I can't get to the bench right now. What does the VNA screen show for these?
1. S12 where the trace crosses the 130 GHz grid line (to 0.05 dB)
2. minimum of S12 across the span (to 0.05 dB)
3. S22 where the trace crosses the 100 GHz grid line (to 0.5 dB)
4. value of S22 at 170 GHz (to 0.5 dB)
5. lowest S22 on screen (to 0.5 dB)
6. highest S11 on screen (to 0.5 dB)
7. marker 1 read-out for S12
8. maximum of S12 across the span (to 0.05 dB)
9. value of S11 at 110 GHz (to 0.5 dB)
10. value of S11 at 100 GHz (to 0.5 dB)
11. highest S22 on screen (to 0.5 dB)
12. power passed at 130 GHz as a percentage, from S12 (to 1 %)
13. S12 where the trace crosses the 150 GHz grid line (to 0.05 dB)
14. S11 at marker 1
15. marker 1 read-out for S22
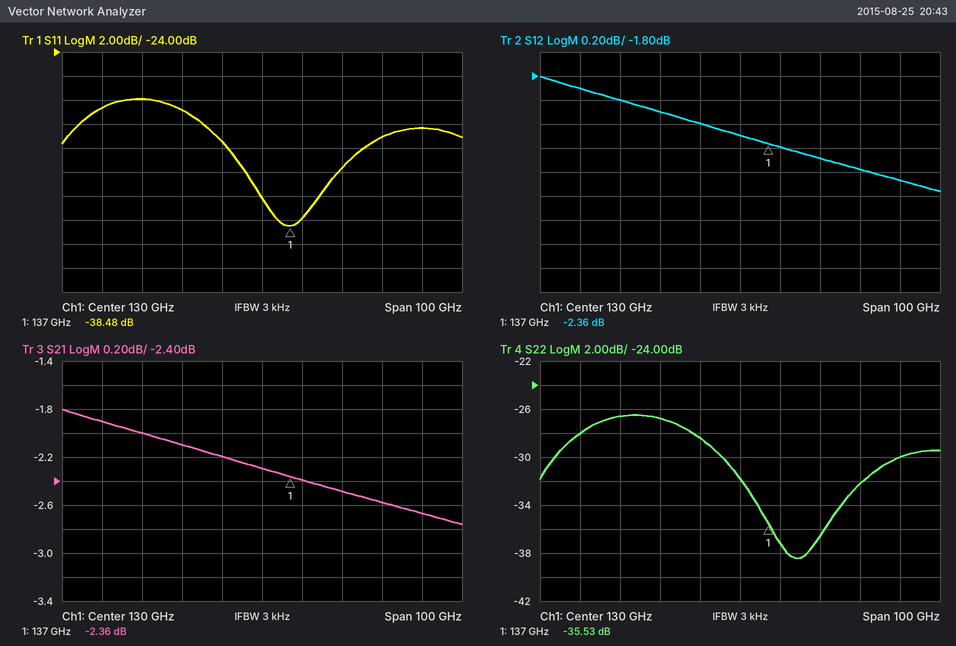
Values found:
-2.30 dB
-2.75 dB
-26.5 dB
-30.0 dB
-38.5 dB
-28.0 dB
-2.36 dB
-1.80 dB
-29.0 dB
-28.0 dB
-26.5 dB
59 %
-2.50 dB
-38.48 dB
-35.53 dB
